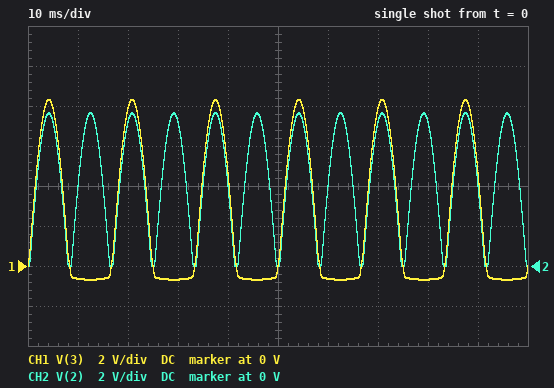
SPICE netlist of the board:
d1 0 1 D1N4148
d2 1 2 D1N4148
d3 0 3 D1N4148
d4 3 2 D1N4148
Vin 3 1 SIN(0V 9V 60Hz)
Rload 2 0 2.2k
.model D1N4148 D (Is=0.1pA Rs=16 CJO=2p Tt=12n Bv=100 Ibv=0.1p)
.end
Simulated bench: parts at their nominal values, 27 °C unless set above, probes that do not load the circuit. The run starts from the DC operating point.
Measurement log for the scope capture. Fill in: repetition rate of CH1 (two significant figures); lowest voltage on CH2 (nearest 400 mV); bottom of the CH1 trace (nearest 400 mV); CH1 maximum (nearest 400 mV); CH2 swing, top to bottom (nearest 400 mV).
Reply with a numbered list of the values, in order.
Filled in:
1. 60 Hz
2. 0 V
3. -800 mV
4. 8.4 V
5. 7.6 V
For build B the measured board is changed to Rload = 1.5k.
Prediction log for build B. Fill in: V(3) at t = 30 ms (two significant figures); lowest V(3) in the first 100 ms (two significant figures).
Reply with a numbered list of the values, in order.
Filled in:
1. -710 mV
2. -720 mV
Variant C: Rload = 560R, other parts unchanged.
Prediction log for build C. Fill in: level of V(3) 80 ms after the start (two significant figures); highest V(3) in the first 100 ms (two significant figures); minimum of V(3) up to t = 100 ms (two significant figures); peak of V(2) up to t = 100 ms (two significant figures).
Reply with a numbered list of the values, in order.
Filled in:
1. -860 mV
2. 8.1 V
3. -870 mV
4. 7.3 V
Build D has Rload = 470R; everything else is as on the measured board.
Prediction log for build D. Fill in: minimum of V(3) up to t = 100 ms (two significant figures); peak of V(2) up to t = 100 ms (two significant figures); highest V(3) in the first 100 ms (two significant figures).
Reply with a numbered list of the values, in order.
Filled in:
1. -910 mV
2. 7.2 V
3. 8.1 V
